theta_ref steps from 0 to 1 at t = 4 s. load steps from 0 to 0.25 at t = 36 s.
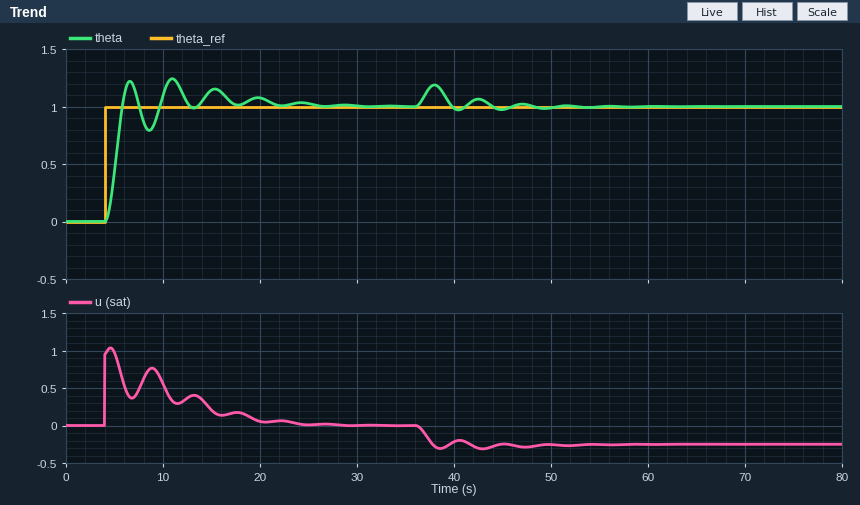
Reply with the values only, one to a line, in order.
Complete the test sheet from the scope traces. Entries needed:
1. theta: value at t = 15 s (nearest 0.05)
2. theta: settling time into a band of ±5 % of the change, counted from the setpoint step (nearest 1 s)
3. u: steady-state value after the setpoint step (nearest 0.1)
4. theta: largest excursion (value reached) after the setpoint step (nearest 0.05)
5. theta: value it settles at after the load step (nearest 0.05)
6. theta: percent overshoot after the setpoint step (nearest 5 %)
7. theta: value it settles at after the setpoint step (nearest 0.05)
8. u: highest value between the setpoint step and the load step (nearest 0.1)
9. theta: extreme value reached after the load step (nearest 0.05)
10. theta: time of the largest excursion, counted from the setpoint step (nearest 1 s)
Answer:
1.15
17 s
0.0
1.25
1.00
25 %
1.00
1.0
1.20
7 s
